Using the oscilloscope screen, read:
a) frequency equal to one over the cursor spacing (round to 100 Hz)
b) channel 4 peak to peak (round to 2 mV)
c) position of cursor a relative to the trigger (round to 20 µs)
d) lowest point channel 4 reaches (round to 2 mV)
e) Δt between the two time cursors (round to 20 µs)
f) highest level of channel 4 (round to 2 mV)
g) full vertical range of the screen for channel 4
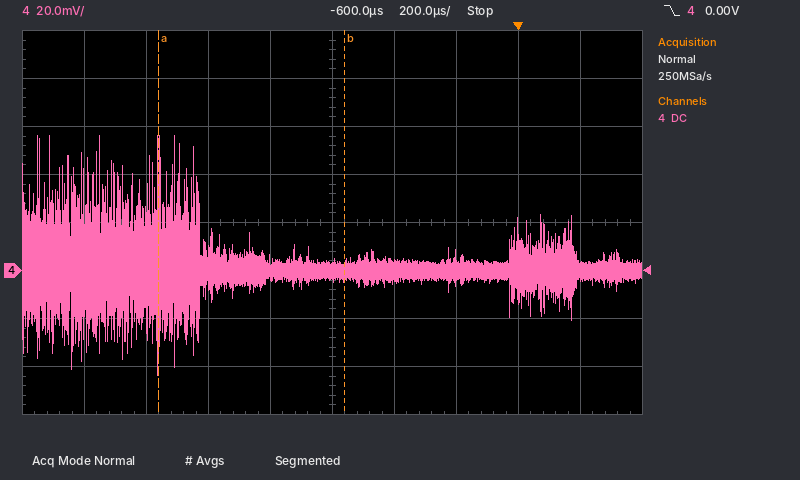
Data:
1.7 kHz
100 mV
-1.16 ms
-44 mV
600 µs
56 mV
160 mV
